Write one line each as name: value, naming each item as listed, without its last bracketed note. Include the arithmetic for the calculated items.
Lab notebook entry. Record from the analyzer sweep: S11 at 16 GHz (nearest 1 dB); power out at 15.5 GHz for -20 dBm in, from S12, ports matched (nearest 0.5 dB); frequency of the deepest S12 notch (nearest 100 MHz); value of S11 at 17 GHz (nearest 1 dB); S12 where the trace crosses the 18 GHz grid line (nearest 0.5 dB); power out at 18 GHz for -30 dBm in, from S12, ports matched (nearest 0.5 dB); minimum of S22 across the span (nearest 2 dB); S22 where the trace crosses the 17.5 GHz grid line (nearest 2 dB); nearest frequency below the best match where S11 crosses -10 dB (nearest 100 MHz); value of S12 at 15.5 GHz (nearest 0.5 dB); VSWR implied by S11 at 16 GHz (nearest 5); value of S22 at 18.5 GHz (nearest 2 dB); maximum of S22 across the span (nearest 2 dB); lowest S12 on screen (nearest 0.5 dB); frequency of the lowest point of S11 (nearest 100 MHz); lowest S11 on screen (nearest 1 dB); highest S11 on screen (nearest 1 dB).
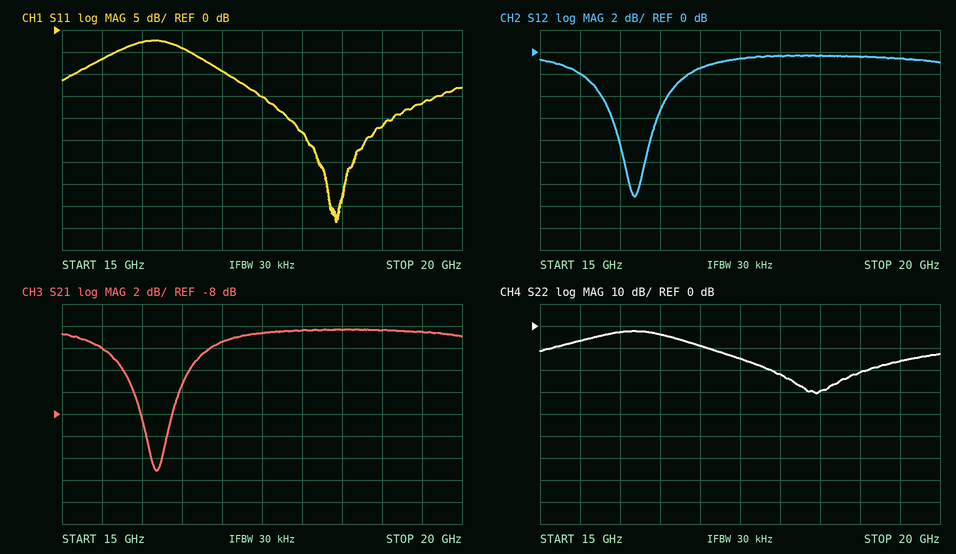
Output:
S11 at 16 GHz: -3 dB
power out at 15.5 GHz for -20 dBm in, from S12, ports matched: -20 dBm + (-2.0 dB) = -22.0 dBm
frequency of the deepest S12 notch: 16.2 GHz
value of S11 at 17 GHz: -9 dB
S12 where the trace crosses the 18 GHz grid line: -0.5 dB
power out at 18 GHz for -30 dBm in, from S12, ports matched: -30 dBm + (-0.5 dB) = -30.5 dBm
minimum of S22 across the span: -30 dB
S22 where the trace crosses the 17.5 GHz grid line: -14 dB
nearest frequency below the best match where S11 crosses -10 dB: 17.1 GHz
value of S12 at 15.5 GHz: -2.0 dB
VSWR implied by S11 at 16 GHz: |Γ| = 10^(-3/20) = 0.7079; VSWR = (1 + 0.7079)/(1 − 0.7079) ≈ 5.85, so 5 to the nearest 5
value of S22 at 18.5 GHz: -30 dB
maximum of S22 across the span: -2 dB
lowest S12 on screen: -13.0 dB
frequency of the lowest point of S11: 18.4 GHz
lowest S11 on screen: -44 dB
highest S11 on screen: -2 dB
